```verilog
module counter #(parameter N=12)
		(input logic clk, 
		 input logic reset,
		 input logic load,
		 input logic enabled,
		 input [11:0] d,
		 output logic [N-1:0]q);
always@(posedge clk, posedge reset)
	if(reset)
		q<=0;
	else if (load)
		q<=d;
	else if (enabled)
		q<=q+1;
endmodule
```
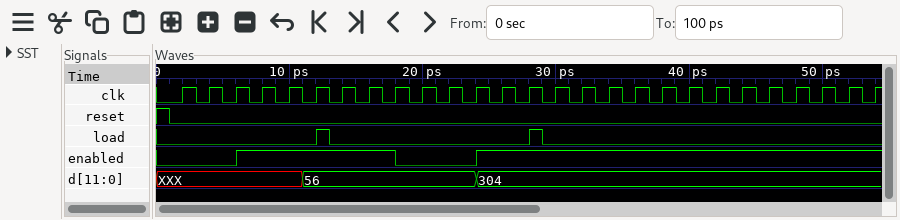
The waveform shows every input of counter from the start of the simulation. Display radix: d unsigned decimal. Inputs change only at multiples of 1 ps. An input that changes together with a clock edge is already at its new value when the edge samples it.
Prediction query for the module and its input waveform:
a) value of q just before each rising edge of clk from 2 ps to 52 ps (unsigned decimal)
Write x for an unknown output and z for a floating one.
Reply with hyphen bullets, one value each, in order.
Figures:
- 0, 0, 0, 1, 2, 3, 56, 57, 58, 58, 58, 58, 59, 60, 304, 305, 306, 307, 308, 309, 310, 311, 312, 313, 314, 315
